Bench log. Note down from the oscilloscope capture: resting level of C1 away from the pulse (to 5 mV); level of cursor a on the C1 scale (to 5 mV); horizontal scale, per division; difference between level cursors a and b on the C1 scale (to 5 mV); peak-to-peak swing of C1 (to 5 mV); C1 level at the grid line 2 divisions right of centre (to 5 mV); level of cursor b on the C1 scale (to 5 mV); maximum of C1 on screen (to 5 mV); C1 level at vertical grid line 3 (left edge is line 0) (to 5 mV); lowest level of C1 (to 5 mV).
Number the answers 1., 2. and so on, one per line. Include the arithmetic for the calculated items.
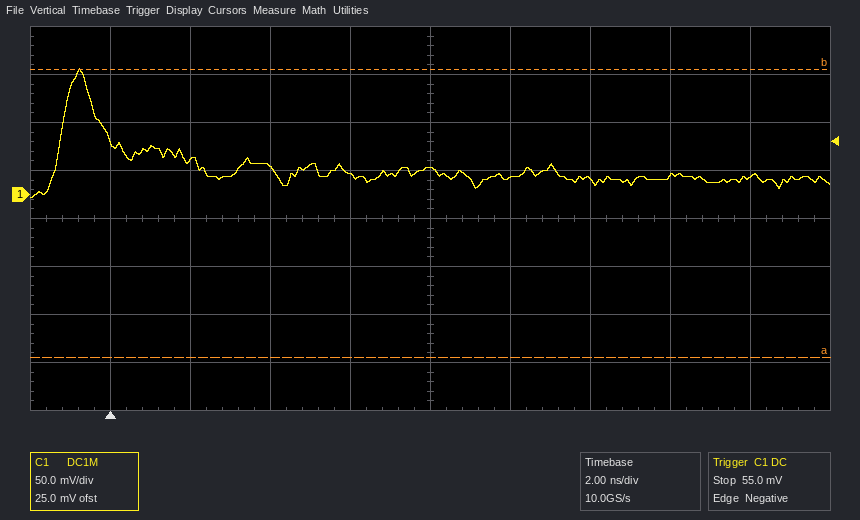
1. 20 mV
2. -170 mV
3. 2 ns
4. 300 mV
5. 130 mV − (-5 mV) = 135 mV
6. 15 mV
7. 130 mV
8. 130 mV
9. 30 mV
10. -5 mV
